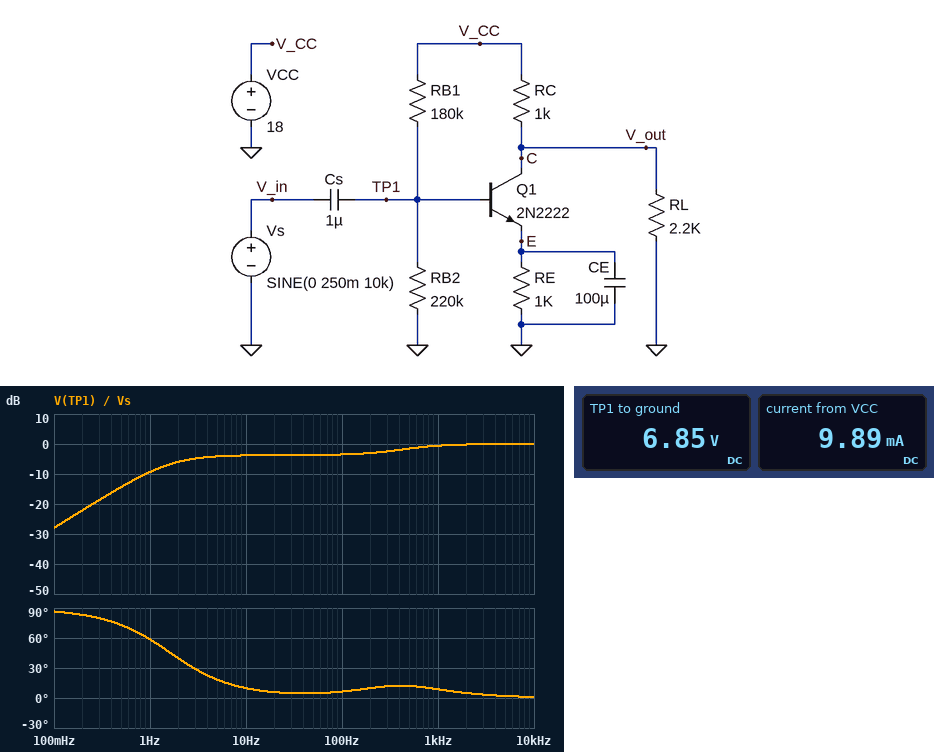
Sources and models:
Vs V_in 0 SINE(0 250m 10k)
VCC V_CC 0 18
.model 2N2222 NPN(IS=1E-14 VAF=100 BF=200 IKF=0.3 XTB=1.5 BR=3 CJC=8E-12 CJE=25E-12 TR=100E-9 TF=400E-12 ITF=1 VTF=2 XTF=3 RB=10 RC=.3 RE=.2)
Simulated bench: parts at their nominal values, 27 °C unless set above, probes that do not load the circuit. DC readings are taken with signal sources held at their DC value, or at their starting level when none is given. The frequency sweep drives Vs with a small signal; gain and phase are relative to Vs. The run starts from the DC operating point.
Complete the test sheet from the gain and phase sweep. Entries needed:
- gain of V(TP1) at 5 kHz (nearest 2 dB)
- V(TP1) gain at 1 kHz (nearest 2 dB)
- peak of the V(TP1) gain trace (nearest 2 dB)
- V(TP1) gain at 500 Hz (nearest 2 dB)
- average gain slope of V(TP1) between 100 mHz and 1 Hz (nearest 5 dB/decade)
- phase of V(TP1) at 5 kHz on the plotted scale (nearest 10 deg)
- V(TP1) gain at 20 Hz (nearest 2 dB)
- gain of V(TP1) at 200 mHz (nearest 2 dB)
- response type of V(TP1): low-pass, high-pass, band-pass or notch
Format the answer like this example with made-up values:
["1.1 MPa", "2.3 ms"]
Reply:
["0 dB", "0 dB", "0 dB", "-2 dB", "20 dB/decade", "0 deg", "-4 dB", "-22 dB", "high-pass"]
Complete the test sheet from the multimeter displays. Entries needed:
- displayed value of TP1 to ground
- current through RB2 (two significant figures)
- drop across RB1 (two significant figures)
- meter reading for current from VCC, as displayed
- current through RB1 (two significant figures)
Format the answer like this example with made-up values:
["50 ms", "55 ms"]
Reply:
["6.85 V", "31 µA", "11 V", "9.89 mA", "62 µA"]
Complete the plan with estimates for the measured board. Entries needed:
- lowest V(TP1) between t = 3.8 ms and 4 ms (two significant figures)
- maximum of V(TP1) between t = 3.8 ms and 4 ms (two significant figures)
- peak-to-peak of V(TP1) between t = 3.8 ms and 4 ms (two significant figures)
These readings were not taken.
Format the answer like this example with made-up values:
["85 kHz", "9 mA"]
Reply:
["6.2 V", "6.7 V", "510 mV"]
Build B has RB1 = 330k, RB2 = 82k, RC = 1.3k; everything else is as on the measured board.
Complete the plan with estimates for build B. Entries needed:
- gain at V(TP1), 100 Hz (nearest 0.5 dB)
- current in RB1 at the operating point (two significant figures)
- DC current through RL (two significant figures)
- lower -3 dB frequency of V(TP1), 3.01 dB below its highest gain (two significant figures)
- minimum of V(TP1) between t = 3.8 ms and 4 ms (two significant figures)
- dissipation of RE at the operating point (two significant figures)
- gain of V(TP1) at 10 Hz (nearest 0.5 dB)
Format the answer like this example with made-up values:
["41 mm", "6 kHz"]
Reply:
["-2.5 dB", "46 µA", "4.3 mA", "57 Hz", "2.4 V", "4.9 mW", "-3.5 dB"]
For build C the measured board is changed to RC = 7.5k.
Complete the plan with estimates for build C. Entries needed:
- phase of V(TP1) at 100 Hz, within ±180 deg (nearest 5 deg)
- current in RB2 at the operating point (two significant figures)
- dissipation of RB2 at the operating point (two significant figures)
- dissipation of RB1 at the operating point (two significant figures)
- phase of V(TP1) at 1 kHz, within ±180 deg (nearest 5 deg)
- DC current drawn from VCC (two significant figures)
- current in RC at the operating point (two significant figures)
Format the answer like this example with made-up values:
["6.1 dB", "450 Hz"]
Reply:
["75 deg", "10 µA", "22 µW", "1.4 mW", "65 deg", "2.3 mA", "2.2 mA"]
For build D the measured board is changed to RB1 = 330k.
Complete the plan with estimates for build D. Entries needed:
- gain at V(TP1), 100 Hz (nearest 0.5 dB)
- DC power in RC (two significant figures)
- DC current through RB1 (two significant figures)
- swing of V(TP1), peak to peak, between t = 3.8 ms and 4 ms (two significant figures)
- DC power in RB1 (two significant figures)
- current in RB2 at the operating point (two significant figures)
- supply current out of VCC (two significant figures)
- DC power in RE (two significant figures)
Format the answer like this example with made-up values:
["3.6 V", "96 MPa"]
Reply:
["-3.0 dB", "70 mW", "40 µA", "500 mV", "540 µW", "21 µA", "8.4 mA", "16 mW"]
